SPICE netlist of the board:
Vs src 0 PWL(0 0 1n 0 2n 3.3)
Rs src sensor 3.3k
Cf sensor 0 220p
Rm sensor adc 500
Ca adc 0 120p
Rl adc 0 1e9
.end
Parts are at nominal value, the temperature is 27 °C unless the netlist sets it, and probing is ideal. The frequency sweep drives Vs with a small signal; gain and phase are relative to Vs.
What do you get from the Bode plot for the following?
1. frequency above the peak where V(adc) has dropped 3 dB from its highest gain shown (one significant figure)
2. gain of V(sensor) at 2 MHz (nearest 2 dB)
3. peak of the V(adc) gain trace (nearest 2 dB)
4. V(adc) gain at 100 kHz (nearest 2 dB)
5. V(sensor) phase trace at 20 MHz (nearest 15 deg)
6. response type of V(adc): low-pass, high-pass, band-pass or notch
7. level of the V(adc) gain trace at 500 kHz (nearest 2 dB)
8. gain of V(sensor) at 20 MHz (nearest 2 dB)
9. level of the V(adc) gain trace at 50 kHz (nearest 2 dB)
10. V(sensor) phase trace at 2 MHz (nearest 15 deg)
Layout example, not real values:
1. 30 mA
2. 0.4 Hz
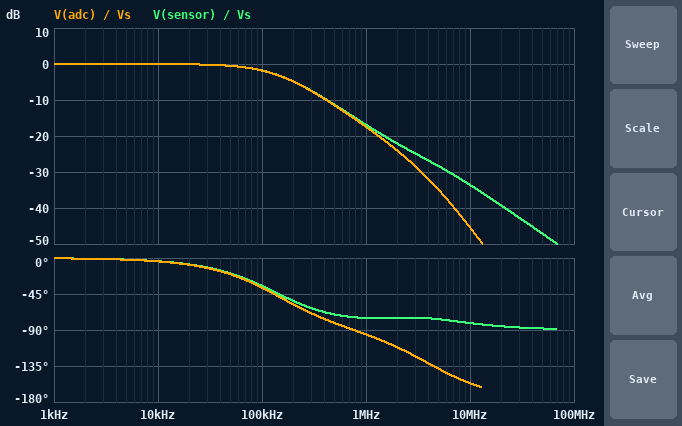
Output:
1. 100 kHz
2. -22 dB
3. 0 dB
4. -2 dB
5. -90 deg
6. low-pass
7. -12 dB
8. -40 dB
9. 0 dB
10. -75 deg
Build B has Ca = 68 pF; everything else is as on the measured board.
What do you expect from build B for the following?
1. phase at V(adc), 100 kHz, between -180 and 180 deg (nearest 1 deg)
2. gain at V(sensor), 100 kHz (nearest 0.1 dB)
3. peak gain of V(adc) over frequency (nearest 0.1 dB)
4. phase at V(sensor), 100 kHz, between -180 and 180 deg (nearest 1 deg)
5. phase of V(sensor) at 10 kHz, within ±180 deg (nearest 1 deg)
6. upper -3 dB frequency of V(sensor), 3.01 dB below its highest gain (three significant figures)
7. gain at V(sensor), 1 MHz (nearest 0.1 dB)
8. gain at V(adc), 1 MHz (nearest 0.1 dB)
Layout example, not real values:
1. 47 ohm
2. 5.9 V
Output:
1. -32 deg
2. -1.3 dB
3. 0 dB
4. -31 deg
5. -3 deg
6. 166 kHz
7. -15.6 dB
8. -15.8 dB
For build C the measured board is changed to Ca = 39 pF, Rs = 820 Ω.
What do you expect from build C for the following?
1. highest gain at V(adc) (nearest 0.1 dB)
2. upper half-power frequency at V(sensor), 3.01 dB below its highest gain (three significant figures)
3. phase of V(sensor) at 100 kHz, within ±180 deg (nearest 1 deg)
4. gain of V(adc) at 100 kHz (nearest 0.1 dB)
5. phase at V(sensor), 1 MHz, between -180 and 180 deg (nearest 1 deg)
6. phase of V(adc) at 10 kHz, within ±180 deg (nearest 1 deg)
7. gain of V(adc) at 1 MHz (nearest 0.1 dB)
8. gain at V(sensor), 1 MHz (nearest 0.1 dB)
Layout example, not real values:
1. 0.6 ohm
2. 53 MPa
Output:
1. 0 dB
2. 740 kHz
3. -8 deg
4. -0.1 dB
5. -52 deg
6. -1 deg
7. -4.6 dB
8. -4.5 dB
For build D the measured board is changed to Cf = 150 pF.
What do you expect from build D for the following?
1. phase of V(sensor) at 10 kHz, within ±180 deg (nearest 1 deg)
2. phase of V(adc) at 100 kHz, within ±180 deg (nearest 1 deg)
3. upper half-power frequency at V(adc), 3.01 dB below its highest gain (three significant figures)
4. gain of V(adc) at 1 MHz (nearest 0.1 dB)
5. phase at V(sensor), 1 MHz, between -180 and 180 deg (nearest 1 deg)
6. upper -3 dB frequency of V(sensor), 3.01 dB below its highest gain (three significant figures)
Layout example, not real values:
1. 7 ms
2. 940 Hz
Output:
1. -3 deg
2. -31 deg
3. 173 kHz
4. -15.5 dB
5. -71 deg
6. 174 kHz
